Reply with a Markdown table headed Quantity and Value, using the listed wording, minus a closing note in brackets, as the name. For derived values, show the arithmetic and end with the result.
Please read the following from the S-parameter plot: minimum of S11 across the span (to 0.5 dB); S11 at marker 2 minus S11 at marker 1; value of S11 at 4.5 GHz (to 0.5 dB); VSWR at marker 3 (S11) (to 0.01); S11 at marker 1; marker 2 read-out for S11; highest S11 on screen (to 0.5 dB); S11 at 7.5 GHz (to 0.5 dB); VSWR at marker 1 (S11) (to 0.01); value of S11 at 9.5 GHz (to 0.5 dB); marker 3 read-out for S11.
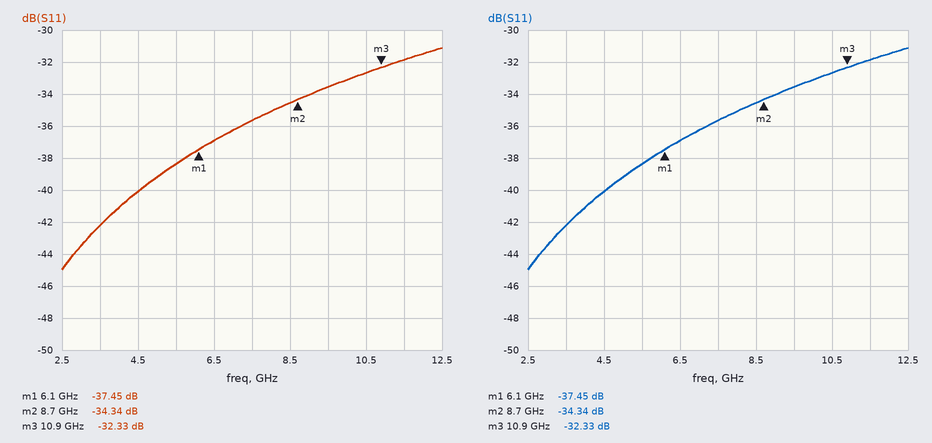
| Quantity | Value |
|---|---|
| minimum of S11 across the span | -45.0 dB |
| S11 at marker 2 minus S11 at marker 1 | -34.34 − (-37.45) = 3.11 dB |
| value of S11 at 4.5 GHz | -40.0 dB |
| VSWR at marker 3 (S11) | (1 + 0.0242)/(1 − 0.0242) ≈ 1.05 |
| S11 at marker 1 | -37.45 dB |
| marker 2 read-out for S11 | -34.34 dB |
| highest S11 on screen | -31.0 dB |
| S11 at 7.5 GHz | -35.5 dB |
| VSWR at marker 1 (S11) | (1 + 0.0134)/(1 − 0.0134) ≈ 1.03 |
| value of S11 at 9.5 GHz | -33.5 dB |
| marker 3 read-out for S11 | -32.33 dB |
